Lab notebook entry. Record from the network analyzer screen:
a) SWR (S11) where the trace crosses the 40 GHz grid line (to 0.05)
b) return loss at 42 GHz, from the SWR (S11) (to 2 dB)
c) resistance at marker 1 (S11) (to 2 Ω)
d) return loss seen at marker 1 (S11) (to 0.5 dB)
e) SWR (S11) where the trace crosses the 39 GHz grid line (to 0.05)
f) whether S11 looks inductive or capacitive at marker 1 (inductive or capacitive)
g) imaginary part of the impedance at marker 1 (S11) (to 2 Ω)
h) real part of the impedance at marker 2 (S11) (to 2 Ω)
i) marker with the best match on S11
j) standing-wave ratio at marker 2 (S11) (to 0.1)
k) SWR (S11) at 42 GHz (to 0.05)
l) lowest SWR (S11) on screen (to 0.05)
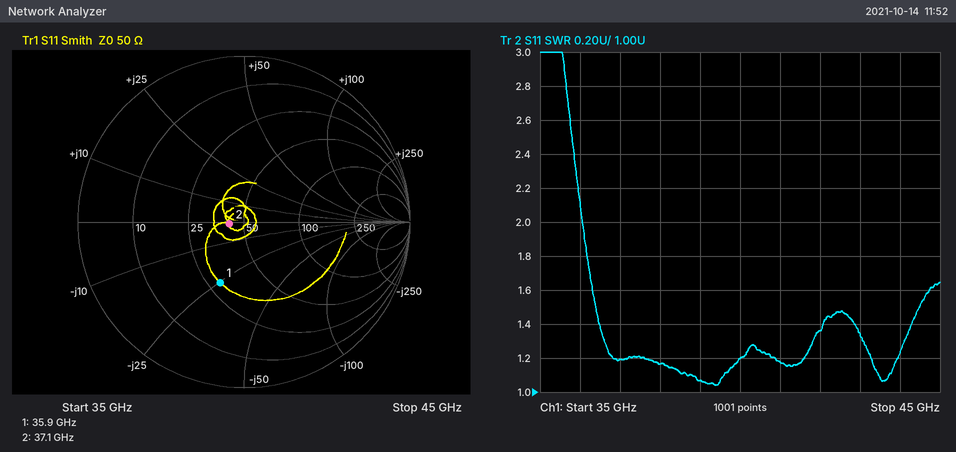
1.20
16 dB
30 Ω
8.0 dB
1.05
capacitive
-26 Ω
42 Ω
marker 2
1.2
1.35
1.05
